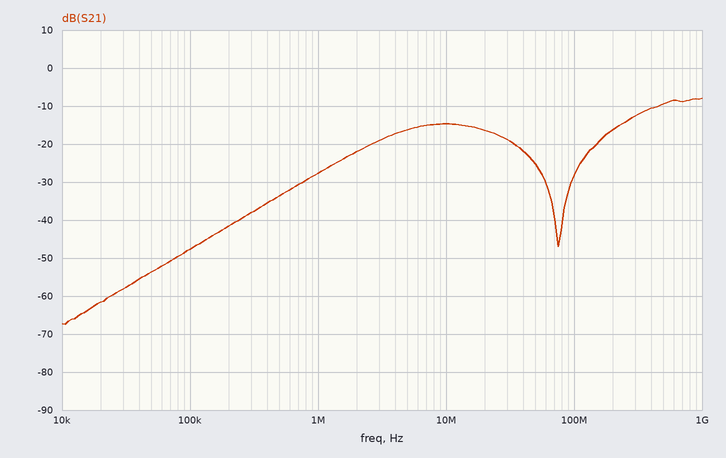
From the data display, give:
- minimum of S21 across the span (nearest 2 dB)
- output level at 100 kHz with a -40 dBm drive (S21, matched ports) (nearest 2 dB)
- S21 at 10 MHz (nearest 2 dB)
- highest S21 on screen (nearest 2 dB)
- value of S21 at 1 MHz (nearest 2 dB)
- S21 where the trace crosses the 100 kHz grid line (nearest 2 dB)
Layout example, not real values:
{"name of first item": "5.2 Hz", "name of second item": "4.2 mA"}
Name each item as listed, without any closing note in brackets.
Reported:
{"minimum of S21 across the span": "-68 dB", "output level at 100 kHz with a -40 dBm drive (S21, matched ports)": "-88 dBm", "S21 at 10 MHz": "-14 dB", "highest S21 on screen": "-8 dB", "value of S21 at 1 MHz": "-28 dB", "S21 where the trace crosses the 100 kHz grid line": "-48 dB"}
